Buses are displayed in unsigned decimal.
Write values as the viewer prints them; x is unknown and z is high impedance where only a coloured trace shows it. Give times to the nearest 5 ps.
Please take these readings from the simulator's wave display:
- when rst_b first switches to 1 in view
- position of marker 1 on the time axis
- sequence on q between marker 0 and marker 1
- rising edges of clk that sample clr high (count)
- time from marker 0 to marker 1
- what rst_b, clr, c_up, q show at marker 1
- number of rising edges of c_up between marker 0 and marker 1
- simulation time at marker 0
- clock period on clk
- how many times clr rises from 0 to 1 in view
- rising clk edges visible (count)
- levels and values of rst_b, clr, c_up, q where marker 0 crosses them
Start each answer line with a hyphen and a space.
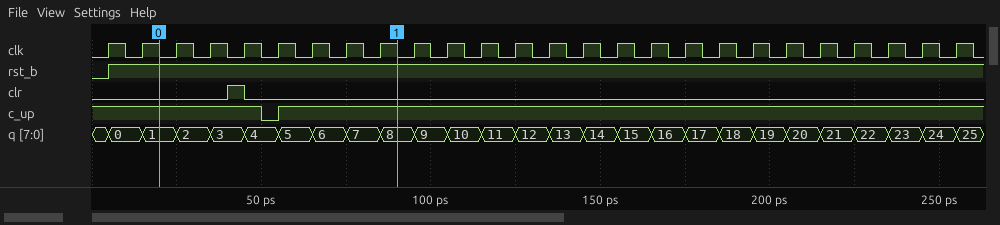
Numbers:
- 5 ps
- 90 ps
- 1, 2, 3, 4, 5, 6, 7, 8
- 1
- 70 ps
- rst_b=1, clr=0, c_up=1, q=8
- 1
- 20 ps
- 10 ps
- 1
- 26
- rst_b=1, clr=0, c_up=1, q=1
